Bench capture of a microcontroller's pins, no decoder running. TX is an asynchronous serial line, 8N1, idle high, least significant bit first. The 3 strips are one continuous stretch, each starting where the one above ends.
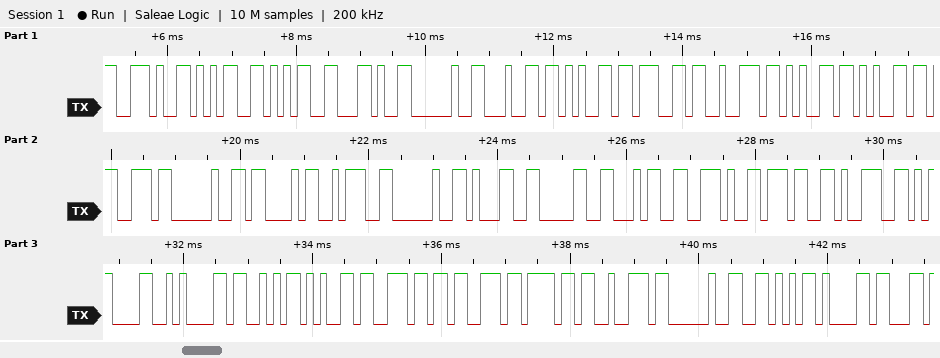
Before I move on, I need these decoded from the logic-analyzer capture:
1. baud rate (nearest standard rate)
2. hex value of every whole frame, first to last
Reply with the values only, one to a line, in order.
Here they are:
9600 baud
2E 35 35 2C 20 64 65 67 72 65 65 73 20 43 3A 20 31 30 34 2E 37 39 0D 0A 53 65 6E 73 6F 72 20 56 61
